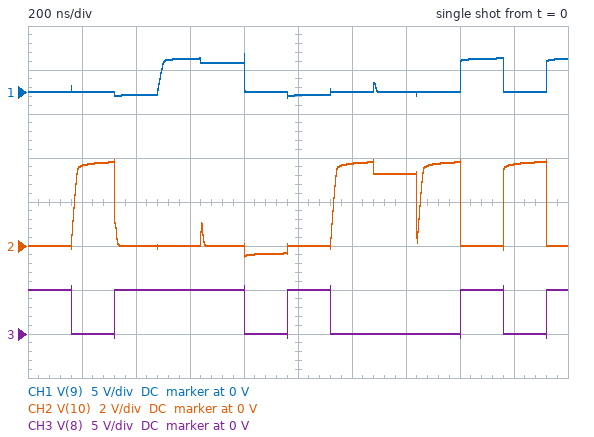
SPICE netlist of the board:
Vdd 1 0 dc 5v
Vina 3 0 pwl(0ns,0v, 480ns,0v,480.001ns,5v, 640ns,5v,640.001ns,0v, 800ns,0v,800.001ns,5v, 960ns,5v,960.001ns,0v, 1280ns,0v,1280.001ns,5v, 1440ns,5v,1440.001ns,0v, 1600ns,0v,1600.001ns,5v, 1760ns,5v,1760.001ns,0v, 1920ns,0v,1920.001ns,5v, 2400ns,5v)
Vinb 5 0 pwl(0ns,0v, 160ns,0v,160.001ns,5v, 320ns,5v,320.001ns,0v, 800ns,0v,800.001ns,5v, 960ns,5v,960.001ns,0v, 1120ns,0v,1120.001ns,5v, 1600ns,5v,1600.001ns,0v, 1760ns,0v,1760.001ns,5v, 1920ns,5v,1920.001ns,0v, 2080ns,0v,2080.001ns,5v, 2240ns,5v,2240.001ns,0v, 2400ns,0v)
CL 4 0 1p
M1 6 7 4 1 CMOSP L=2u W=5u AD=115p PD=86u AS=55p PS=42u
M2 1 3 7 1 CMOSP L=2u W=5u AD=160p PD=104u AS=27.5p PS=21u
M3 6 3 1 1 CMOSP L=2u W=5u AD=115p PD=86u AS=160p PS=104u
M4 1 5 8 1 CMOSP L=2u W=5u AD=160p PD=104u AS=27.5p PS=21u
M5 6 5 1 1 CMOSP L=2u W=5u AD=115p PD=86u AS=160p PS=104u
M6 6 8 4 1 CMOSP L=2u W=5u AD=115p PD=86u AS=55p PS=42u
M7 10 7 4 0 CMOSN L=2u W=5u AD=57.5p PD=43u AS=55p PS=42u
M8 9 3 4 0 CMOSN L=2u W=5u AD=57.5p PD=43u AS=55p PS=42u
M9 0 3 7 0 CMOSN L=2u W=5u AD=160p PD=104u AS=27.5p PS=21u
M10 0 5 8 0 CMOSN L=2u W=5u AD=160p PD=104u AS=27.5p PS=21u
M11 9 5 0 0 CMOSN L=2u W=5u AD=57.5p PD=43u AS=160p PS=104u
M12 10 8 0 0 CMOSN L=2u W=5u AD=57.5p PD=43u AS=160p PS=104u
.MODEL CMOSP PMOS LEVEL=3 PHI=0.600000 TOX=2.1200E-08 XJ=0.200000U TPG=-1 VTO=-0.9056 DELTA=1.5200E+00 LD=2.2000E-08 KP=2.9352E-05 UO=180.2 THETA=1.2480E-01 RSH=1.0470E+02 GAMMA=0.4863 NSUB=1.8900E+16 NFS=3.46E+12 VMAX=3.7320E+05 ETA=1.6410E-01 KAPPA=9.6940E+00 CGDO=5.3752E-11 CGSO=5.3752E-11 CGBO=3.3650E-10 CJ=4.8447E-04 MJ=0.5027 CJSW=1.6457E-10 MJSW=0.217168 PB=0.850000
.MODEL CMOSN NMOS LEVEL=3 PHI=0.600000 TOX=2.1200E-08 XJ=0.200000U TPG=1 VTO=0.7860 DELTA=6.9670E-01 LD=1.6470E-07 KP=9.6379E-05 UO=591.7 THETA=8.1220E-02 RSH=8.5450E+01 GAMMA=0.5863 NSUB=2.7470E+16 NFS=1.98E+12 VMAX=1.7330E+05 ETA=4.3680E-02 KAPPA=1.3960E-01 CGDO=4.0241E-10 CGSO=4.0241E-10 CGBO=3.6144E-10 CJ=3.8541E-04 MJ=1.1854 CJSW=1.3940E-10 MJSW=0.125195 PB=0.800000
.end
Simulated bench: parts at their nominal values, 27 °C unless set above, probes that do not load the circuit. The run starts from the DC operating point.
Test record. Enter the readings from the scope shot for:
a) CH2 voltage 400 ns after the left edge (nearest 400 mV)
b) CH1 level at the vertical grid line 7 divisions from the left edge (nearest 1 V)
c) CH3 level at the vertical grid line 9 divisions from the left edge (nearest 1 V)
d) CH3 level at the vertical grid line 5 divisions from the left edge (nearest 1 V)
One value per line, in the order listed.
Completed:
0 V
0 V
0 V
5 V
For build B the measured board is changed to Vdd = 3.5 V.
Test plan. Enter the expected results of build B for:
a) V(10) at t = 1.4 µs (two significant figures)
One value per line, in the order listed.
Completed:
2.2 V
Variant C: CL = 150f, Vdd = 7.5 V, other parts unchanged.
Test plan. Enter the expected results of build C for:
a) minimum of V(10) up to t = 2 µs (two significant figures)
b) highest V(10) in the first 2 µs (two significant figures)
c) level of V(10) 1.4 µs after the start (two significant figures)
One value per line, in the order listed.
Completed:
-480 mV
6.2 V
5.2 V
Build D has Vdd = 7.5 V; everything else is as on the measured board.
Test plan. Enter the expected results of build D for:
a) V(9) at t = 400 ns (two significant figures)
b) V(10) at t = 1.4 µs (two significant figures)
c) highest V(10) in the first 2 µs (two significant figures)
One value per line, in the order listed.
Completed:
-360 mV
5.2 V
6.2 V
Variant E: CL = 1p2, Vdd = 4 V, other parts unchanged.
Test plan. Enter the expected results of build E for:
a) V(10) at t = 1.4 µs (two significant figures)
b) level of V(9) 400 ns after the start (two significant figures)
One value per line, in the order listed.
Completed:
2.5 V
-360 mV
